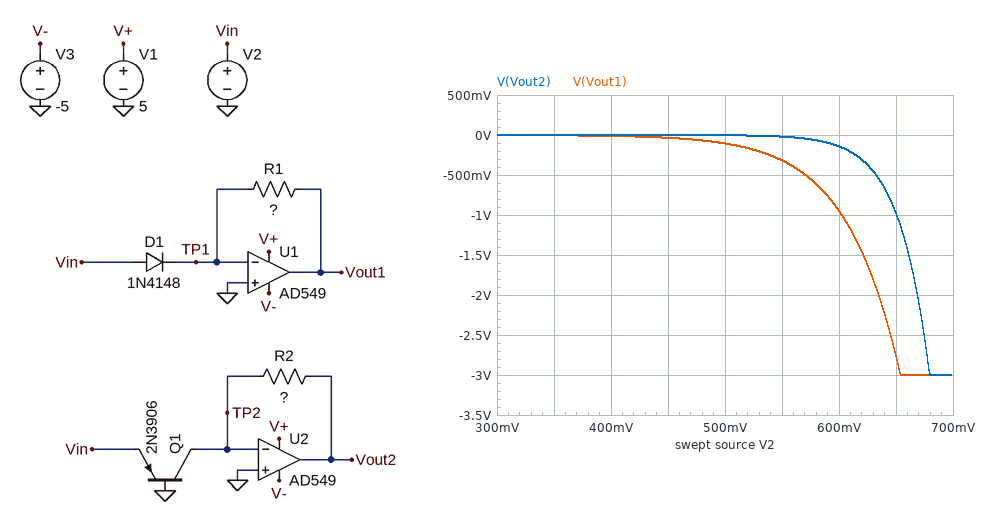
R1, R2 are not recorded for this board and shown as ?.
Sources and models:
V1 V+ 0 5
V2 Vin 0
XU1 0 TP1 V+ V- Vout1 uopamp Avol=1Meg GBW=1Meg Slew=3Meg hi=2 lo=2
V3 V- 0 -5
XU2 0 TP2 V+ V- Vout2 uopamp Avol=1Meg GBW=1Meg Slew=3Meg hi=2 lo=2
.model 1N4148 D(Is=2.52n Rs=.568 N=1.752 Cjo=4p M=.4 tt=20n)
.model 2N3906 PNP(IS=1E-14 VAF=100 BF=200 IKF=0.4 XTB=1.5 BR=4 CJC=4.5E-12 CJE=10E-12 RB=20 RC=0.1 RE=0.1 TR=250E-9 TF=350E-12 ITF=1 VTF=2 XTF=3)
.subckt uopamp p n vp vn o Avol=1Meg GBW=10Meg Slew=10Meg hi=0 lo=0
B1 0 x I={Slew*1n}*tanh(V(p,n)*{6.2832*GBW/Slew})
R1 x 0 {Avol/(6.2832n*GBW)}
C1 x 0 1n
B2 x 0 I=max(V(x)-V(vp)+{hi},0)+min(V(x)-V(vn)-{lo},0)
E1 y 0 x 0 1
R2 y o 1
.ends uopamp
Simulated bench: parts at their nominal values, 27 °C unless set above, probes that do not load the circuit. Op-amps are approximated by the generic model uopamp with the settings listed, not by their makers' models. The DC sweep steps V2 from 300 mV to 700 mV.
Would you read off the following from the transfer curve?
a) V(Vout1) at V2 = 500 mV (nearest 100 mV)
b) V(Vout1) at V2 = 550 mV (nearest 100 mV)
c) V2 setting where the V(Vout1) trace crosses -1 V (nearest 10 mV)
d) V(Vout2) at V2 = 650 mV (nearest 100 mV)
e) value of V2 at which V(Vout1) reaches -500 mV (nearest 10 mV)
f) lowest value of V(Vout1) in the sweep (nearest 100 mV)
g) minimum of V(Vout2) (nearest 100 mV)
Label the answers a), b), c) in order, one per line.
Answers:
a) -100 mV
b) -300 mV
c) 600 mV
d) -1.0 V
e) 570 mV
f) -3.0 V
g) -3.0 V
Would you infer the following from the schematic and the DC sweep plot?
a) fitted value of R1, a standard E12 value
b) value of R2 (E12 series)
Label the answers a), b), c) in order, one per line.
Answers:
a) 680 Ω
b) 1.2 kΩ
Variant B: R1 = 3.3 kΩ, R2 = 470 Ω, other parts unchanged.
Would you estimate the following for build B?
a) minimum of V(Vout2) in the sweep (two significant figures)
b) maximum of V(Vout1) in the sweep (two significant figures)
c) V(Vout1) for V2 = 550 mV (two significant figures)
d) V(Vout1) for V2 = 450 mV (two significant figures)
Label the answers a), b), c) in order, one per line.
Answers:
a) -2.5 V
b) -6.2 mV
c) -1.5 V
d) -170 mV
